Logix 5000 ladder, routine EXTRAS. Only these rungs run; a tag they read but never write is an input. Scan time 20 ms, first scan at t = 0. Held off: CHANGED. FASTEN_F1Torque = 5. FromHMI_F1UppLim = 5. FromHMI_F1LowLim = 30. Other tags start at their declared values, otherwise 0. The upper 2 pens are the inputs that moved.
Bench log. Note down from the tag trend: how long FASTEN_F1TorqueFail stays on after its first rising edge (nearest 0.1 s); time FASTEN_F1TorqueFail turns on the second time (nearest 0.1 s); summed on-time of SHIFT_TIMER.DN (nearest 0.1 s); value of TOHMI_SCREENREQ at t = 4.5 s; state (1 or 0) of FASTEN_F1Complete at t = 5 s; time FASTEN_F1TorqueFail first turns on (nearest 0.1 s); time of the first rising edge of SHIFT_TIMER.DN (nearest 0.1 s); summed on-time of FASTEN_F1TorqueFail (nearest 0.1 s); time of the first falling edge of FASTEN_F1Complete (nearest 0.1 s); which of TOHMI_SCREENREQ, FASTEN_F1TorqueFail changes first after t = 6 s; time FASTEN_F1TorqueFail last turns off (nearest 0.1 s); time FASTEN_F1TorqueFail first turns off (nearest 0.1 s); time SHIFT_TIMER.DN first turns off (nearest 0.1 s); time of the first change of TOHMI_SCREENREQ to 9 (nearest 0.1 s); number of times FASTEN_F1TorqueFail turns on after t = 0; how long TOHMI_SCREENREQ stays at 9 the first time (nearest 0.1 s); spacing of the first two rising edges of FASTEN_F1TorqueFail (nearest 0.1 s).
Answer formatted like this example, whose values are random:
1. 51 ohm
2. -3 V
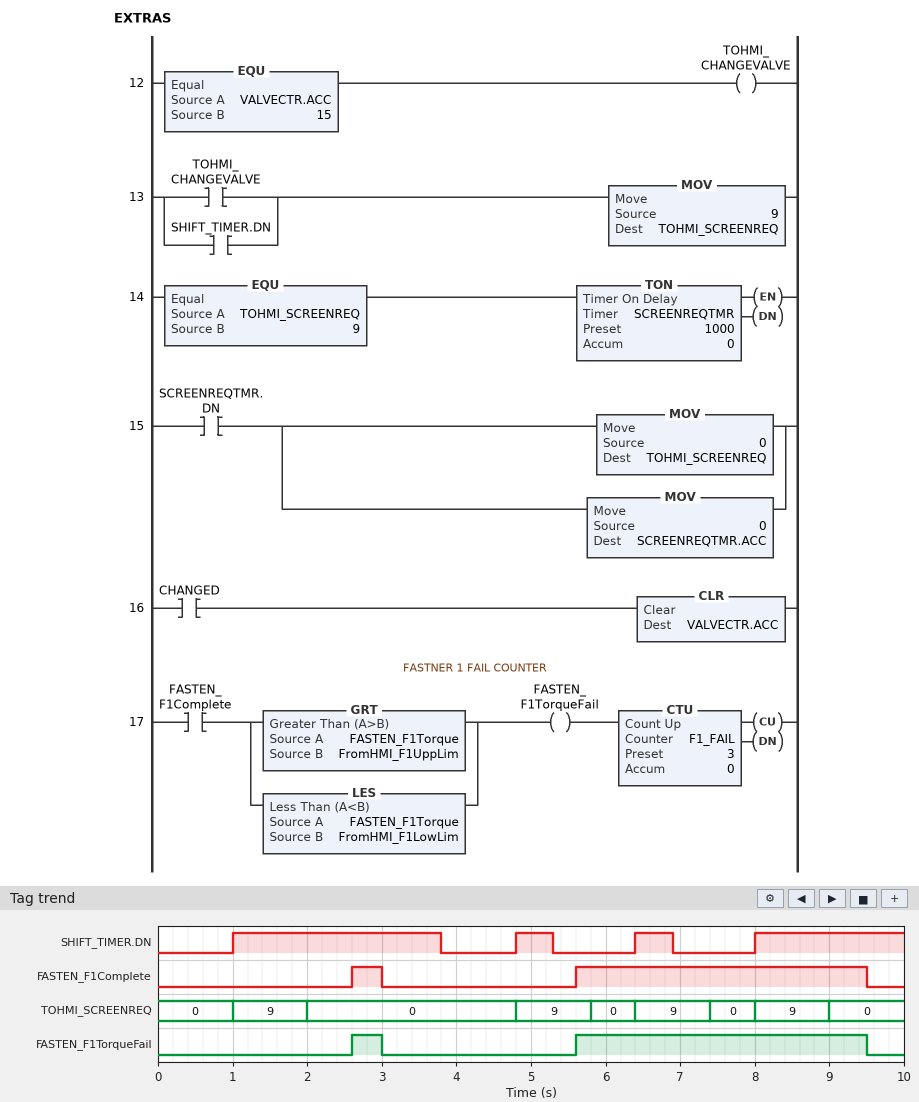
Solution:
1. 0.4 s
2. 5.6 s
3. 5.8 s
4. 0
5. 0
6. 2.6 s
7. 1.0 s
8. 4.3 s
9. 3.0 s
10. TOHMI_SCREENREQ
11. 9.5 s
12. 3.0 s
13. 3.8 s
14. 1.0 s
15. 2
16. 1.0 s
17. 3.0 s
